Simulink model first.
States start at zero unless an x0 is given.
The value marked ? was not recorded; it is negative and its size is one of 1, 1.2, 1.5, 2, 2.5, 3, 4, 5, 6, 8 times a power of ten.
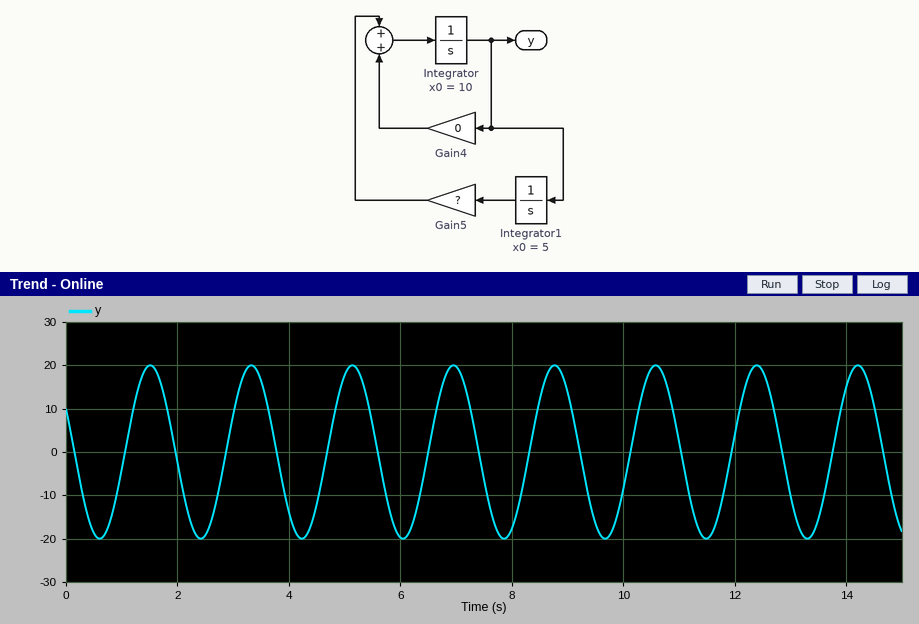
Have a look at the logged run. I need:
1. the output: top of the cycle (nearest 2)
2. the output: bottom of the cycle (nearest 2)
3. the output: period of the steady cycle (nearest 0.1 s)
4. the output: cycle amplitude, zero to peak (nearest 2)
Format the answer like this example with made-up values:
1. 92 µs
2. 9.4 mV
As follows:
1. 20
2. -20
3. 1.8 s
4. 20
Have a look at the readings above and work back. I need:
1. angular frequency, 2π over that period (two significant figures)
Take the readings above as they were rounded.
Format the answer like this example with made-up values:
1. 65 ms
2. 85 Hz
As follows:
1. 3.5 rad/s
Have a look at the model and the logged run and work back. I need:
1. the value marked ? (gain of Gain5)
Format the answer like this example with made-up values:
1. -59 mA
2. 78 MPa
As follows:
1. -12
